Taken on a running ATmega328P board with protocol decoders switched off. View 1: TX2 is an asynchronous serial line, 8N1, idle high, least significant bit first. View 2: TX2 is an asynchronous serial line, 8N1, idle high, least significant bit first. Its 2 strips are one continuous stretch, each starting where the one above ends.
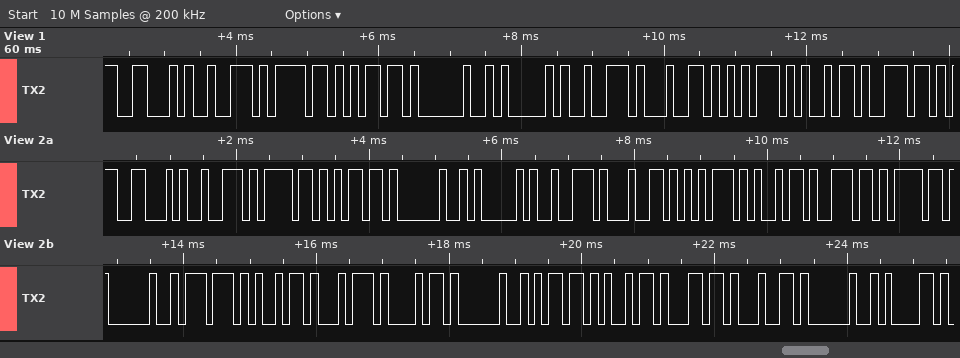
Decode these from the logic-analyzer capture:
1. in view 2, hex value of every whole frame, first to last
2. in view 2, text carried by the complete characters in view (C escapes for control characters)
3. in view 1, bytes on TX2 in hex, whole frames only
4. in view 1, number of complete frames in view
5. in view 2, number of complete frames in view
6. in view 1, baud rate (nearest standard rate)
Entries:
46 72 6F 6D 20 41 72 64 75 69 6E 6F 20 77 69 74 68 20 6D 69 6C 64 20 61
"From Arduino with mild a"
46 72 6F 6D 20 41 72 64 75 69 6E
11
24
9600 baud
